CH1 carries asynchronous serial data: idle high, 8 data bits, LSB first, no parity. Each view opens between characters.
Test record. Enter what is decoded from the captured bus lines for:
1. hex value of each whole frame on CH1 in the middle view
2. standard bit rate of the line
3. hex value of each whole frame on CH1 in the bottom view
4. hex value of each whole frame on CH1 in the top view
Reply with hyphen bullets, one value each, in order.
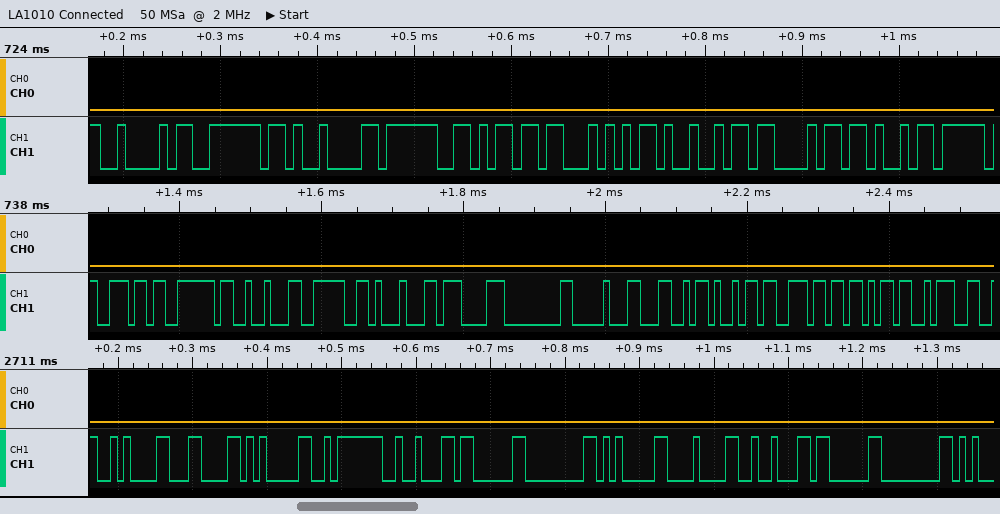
- 6E, 7E, 12, 3E, 11, 87, 00, 10, 4C, 69, 6E, 6B, 3A
- 115200 baud
- 0A, 0C, 05, FA, 12, 03, 00, 05, 08, 12, 03, 00
- 42, 7E, 09, 3F, 6D, 54, 49, 43, 4B
